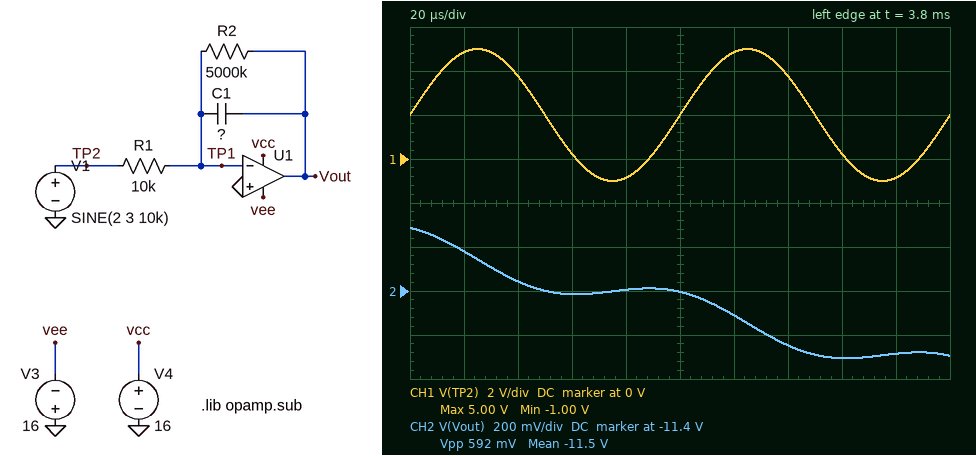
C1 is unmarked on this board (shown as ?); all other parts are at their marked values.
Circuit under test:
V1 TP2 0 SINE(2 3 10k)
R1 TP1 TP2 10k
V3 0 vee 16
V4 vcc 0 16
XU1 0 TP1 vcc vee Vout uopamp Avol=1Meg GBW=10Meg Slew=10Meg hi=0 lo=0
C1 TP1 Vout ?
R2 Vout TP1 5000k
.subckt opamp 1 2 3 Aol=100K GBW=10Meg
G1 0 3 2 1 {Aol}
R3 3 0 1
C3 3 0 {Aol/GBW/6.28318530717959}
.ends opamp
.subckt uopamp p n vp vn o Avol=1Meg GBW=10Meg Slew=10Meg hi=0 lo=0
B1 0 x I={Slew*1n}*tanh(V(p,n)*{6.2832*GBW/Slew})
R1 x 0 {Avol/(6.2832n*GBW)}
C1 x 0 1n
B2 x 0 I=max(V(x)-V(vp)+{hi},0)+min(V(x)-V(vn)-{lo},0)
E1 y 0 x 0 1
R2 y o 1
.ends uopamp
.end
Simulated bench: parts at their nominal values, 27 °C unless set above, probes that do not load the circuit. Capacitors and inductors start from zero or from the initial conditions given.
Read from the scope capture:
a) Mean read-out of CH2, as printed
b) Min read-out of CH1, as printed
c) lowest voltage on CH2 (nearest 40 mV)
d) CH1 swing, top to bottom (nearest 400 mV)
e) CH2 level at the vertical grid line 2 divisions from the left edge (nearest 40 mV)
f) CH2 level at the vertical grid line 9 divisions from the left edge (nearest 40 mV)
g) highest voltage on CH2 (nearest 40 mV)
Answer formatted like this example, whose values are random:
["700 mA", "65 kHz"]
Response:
["-11.5 V", "-1.00 V", "-11.72 V", "6.0 V", "-11.36 V", "-11.68 V", "-11.12 V"]
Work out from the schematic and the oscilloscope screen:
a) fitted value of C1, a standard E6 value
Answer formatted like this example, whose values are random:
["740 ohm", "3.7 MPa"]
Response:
["68 nF"]
